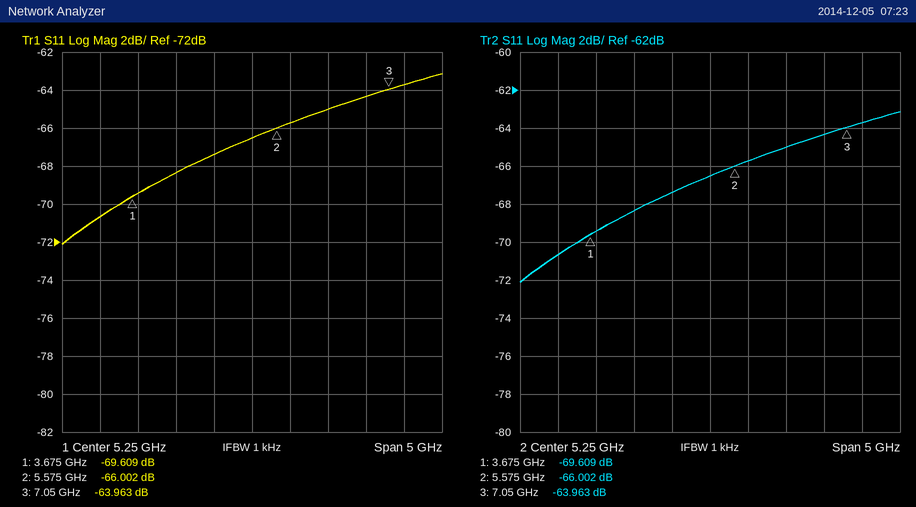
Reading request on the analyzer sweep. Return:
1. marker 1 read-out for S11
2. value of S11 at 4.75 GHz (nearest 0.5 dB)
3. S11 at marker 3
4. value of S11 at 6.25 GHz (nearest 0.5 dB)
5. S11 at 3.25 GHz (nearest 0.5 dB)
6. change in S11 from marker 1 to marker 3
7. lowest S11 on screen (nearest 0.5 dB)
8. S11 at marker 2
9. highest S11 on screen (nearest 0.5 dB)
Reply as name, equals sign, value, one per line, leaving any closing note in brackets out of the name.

marker 1 read-out for S11 = -69.609 dB
value of S11 at 4.75 GHz = -67.5 dB
S11 at marker 3 = -63.963 dB
value of S11 at 6.25 GHz = -65.0 dB
S11 at 3.25 GHz = -70.5 dB
change in S11 from marker 1 to marker 3 = 5.646 dB
lowest S11 on screen = -72.0 dB
S11 at marker 2 = -66.002 dB
highest S11 on screen = -63.0 dB
